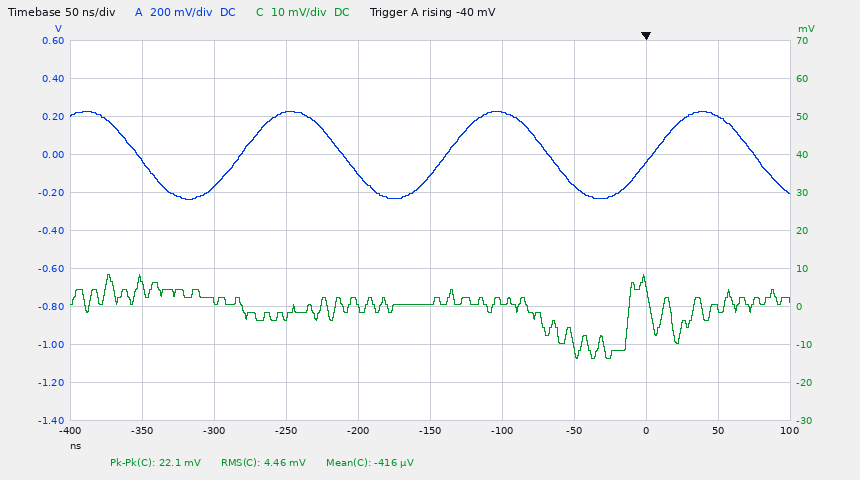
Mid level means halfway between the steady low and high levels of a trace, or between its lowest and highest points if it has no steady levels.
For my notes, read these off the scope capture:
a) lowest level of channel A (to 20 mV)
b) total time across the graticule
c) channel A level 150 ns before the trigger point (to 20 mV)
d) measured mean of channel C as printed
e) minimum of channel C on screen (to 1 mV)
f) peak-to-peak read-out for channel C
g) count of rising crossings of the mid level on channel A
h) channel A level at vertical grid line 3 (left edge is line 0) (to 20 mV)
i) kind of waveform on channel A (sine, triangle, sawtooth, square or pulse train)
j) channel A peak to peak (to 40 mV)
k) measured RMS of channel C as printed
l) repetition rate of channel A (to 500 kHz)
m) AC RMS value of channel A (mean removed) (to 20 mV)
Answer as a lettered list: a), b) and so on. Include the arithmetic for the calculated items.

a) -240 mV
b) 500 ns
c) -120 mV
d) -416 µV
e) -14 mV
f) 22.1 mV
g) 3
h) 220 mV
i) sine
j) 480 mV
k) 4.46 mV
l) 7.0 MHz
m) 480 mV / (2√2) ≈ 170 mV, so 160 mV to the nearest 20 mV
